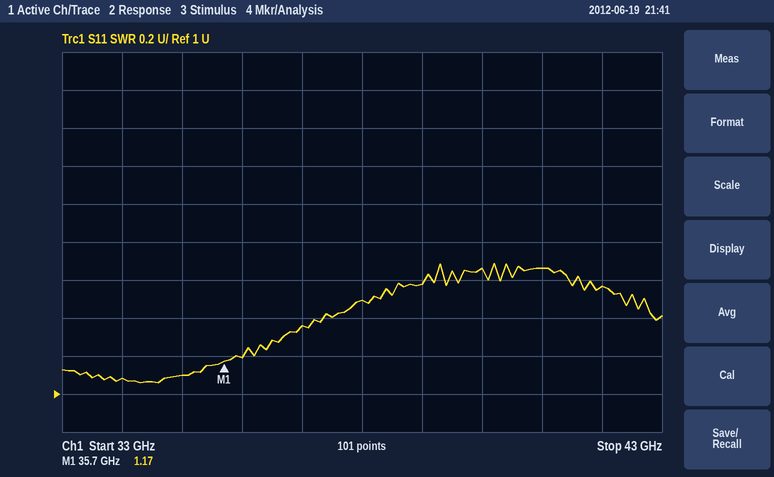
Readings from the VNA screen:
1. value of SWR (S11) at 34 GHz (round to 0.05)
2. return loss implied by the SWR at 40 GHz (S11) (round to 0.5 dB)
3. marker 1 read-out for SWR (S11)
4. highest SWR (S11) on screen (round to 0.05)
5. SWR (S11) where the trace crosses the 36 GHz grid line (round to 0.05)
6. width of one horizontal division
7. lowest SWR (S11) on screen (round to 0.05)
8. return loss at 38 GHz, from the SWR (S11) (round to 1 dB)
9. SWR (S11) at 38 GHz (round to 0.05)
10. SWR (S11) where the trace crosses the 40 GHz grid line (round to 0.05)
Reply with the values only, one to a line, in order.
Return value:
1.10
12.0 dB
1.17
1.70
1.20
1 GHz
1.05
14 dB
1.50
1.65
